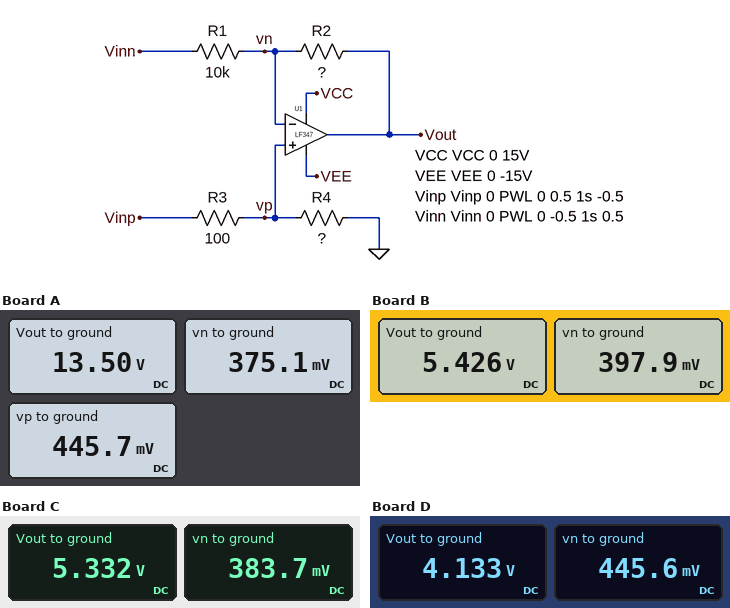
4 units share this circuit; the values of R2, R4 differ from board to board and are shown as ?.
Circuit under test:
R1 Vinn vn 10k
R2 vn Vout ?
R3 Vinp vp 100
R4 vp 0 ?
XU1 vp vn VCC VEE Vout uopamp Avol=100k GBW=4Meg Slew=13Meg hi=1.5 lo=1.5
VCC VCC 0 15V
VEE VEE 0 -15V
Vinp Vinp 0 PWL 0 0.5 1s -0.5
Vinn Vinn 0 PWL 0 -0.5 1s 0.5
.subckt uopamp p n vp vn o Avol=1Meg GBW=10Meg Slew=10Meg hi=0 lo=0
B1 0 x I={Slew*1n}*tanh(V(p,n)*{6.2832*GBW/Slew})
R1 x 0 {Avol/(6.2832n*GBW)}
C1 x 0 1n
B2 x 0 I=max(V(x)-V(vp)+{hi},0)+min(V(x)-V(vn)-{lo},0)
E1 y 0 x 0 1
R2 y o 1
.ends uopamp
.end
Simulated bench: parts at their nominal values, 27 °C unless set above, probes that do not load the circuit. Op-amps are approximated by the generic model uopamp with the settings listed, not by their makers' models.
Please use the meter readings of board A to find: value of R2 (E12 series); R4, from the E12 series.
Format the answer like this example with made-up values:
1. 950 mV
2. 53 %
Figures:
1. 150 kΩ
2. 820 Ω
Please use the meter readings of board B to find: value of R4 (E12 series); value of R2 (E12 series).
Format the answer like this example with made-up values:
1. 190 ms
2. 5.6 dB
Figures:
1. 390 Ω
2. 56 kΩ
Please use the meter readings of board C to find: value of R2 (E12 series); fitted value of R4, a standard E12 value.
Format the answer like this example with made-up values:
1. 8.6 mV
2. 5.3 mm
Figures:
1. 56 kΩ
2. 330 Ω
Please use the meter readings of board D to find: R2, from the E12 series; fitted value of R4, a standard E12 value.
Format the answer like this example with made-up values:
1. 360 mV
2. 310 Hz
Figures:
1. 39 kΩ
2. 820 Ω
